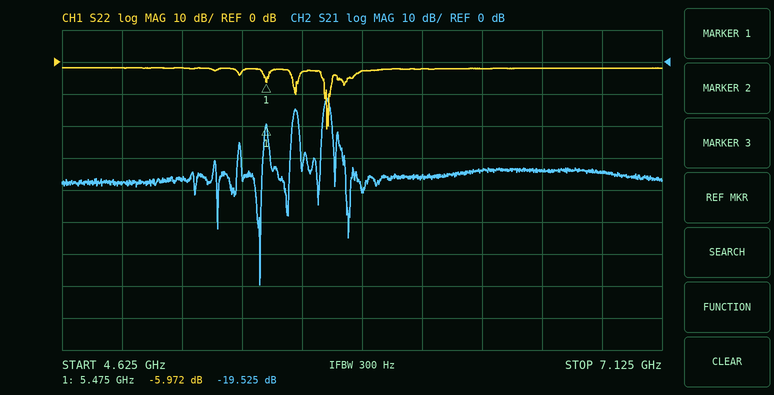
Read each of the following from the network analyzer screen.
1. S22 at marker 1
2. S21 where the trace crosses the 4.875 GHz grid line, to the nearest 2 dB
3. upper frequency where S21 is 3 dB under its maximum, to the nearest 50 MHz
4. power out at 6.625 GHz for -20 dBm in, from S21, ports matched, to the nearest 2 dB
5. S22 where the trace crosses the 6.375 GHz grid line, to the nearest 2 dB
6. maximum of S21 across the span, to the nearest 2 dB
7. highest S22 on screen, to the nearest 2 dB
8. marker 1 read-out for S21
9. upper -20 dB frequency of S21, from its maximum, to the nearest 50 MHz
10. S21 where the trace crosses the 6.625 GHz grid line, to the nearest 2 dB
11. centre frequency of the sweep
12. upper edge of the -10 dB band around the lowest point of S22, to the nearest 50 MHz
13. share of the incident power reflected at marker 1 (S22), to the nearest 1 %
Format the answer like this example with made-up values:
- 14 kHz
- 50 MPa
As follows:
- -5.972 dB
- -38 dB
- 5.75 GHz
- -54 dBm
- -2 dB
- -12 dB
- -2 dB
- -19.525 dB
- 5.75 GHz
- -34 dB
- 5.875 GHz
- 5.75 GHz
- 25 %
